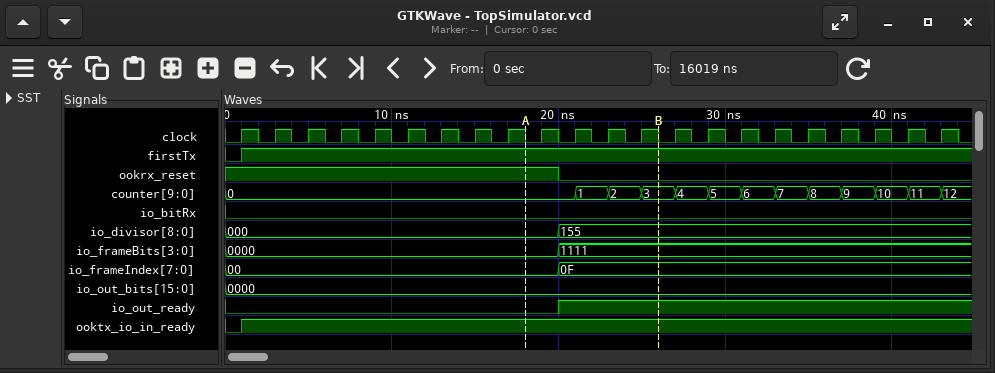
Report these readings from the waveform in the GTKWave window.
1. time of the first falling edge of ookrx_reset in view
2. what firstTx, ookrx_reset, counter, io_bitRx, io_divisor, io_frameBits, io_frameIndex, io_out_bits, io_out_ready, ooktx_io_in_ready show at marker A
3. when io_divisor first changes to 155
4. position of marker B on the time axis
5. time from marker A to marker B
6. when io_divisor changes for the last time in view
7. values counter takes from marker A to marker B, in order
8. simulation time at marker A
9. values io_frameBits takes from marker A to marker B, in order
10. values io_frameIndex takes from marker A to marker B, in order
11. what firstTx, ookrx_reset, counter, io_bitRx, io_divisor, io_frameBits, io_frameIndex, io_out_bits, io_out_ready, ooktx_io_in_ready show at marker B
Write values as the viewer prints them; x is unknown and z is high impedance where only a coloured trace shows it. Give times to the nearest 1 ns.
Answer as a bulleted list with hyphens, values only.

- 20 ns
- firstTx=1, ookrx_reset=1, counter=0, io_bitRx=0, io_divisor=000, io_frameBits=0000, io_frameIndex=00, io_out_bits=0000, io_out_ready=0, ooktx_io_in_ready=1
- 20 ns
- 26 ns
- 8 ns
- 20 ns
- 0, 1, 2, 3
- 18 ns
- 0000, 1111
- 00, 0F
- firstTx=1, ookrx_reset=0, counter=3, io_bitRx=0, io_divisor=155, io_frameBits=1111, io_frameIndex=0F, io_out_bits=0000, io_out_ready=1, ooktx_io_in_ready=1
